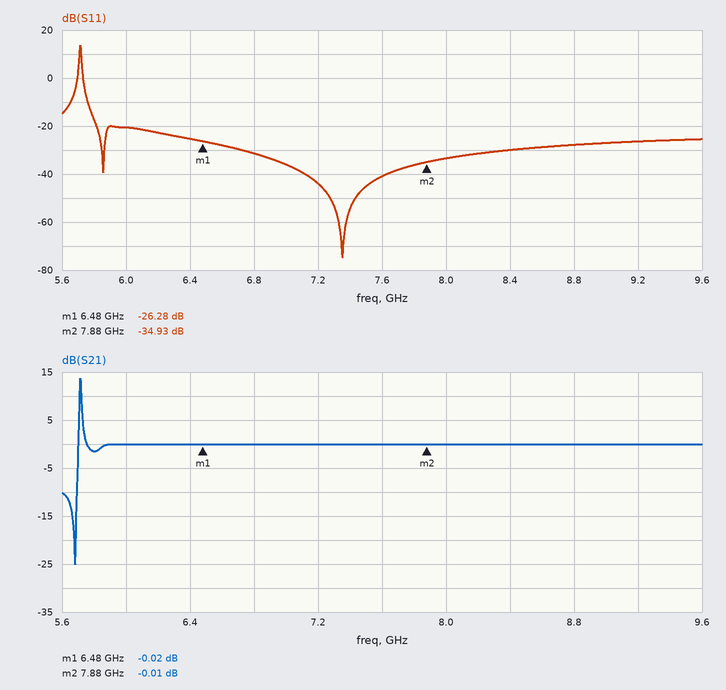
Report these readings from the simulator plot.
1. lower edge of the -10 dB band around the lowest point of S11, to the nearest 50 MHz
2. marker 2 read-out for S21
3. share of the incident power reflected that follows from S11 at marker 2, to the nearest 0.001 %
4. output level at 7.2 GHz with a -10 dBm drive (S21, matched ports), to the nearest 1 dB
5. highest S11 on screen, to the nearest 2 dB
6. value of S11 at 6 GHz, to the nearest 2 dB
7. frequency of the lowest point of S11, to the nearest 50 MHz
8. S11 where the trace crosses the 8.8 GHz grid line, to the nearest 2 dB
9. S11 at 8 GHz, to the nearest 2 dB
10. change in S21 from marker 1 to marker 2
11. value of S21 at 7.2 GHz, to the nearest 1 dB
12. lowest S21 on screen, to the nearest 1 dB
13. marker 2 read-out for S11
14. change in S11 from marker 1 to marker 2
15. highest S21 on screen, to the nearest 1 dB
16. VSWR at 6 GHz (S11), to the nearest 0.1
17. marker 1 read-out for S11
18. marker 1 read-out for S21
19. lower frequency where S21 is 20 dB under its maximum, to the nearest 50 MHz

5.75 GHz
-0.01 dB
0.032 %
-10 dBm
14 dB
-20 dB
7.35 GHz
-28 dB
-34 dB
0.01 dB
0 dB
-25 dB
-34.93 dB
-8.65 dB
14 dB
1.2
-26.28 dB
-0.02 dB
5.70 GHz
